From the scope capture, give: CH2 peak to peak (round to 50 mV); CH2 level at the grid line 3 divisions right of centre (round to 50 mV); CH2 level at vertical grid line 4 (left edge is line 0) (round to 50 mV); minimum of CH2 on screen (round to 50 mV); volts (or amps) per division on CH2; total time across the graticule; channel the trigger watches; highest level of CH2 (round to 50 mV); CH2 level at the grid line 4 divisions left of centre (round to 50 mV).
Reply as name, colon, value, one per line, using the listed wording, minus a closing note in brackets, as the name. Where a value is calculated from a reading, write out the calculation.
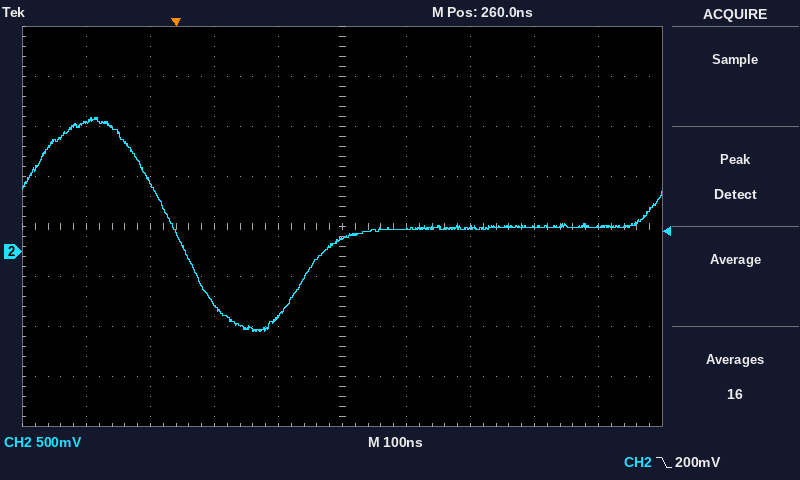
CH2 peak to peak: 1.35 V − (-800 mV) = 2.15 V
CH2 level at the grid line 3 divisions right of centre: 250 mV
CH2 level at vertical grid line 4 (left edge is line 0): -650 mV
minimum of CH2 on screen: -800 mV
volts (or amps) per division on CH2: 500 mV
total time across the graticule: 1 µs
channel the trigger watches: CH2
highest level of CH2: 1.35 V
CH2 level at the grid line 4 divisions left of centre: 1.30 V
